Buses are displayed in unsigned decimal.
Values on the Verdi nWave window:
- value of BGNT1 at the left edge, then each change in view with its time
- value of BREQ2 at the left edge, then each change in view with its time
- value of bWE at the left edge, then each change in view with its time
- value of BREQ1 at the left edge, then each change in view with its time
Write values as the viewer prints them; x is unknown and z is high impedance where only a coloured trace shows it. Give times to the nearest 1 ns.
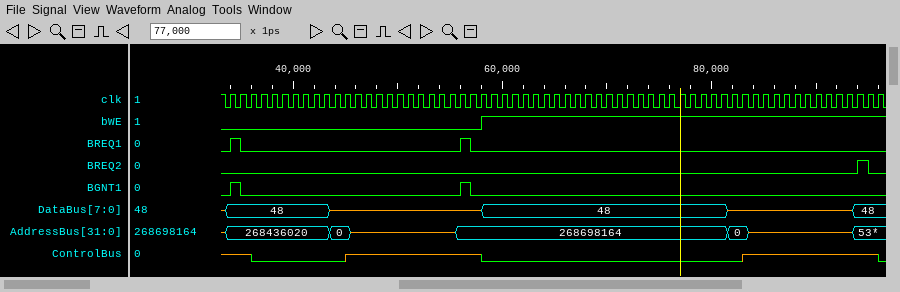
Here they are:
0, 1 at 34 ns, 0 at 35 ns, 1 at 56 ns, 0 at 57 ns
0, 1 at 94 ns, 0 at 95 ns
0, 1 at 58 ns
0, 1 at 34 ns, 0 at 35 ns, 1 at 56 ns, 0 at 57 ns
